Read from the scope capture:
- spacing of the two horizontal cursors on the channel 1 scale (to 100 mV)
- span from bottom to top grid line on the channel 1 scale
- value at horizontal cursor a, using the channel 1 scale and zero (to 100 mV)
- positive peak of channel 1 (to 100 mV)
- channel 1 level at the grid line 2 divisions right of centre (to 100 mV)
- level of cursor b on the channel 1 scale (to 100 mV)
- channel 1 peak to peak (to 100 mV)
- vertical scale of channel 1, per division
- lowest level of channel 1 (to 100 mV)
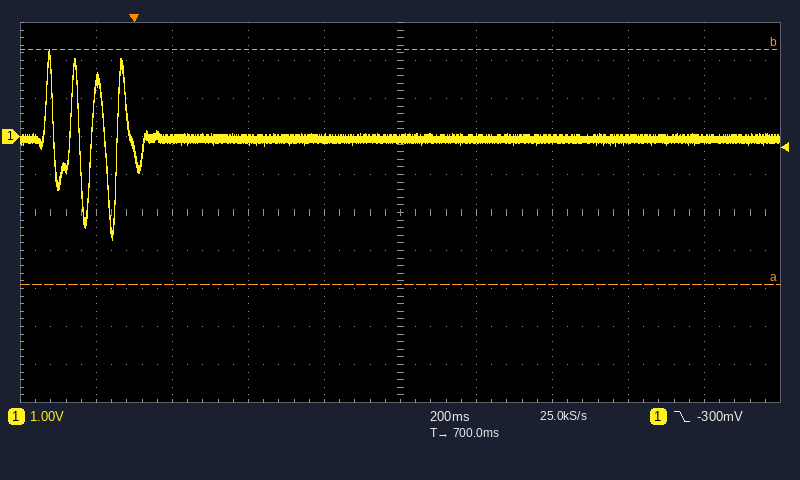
6.2 V
10 V
-3.9 V
2.3 V
-100 mV
2.3 V
5.0 V
1 V
-2.7 V
